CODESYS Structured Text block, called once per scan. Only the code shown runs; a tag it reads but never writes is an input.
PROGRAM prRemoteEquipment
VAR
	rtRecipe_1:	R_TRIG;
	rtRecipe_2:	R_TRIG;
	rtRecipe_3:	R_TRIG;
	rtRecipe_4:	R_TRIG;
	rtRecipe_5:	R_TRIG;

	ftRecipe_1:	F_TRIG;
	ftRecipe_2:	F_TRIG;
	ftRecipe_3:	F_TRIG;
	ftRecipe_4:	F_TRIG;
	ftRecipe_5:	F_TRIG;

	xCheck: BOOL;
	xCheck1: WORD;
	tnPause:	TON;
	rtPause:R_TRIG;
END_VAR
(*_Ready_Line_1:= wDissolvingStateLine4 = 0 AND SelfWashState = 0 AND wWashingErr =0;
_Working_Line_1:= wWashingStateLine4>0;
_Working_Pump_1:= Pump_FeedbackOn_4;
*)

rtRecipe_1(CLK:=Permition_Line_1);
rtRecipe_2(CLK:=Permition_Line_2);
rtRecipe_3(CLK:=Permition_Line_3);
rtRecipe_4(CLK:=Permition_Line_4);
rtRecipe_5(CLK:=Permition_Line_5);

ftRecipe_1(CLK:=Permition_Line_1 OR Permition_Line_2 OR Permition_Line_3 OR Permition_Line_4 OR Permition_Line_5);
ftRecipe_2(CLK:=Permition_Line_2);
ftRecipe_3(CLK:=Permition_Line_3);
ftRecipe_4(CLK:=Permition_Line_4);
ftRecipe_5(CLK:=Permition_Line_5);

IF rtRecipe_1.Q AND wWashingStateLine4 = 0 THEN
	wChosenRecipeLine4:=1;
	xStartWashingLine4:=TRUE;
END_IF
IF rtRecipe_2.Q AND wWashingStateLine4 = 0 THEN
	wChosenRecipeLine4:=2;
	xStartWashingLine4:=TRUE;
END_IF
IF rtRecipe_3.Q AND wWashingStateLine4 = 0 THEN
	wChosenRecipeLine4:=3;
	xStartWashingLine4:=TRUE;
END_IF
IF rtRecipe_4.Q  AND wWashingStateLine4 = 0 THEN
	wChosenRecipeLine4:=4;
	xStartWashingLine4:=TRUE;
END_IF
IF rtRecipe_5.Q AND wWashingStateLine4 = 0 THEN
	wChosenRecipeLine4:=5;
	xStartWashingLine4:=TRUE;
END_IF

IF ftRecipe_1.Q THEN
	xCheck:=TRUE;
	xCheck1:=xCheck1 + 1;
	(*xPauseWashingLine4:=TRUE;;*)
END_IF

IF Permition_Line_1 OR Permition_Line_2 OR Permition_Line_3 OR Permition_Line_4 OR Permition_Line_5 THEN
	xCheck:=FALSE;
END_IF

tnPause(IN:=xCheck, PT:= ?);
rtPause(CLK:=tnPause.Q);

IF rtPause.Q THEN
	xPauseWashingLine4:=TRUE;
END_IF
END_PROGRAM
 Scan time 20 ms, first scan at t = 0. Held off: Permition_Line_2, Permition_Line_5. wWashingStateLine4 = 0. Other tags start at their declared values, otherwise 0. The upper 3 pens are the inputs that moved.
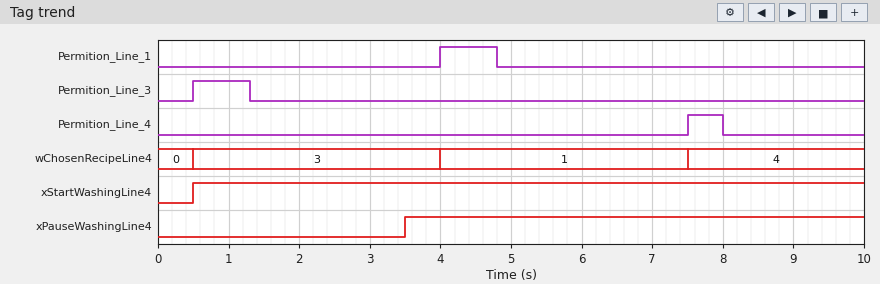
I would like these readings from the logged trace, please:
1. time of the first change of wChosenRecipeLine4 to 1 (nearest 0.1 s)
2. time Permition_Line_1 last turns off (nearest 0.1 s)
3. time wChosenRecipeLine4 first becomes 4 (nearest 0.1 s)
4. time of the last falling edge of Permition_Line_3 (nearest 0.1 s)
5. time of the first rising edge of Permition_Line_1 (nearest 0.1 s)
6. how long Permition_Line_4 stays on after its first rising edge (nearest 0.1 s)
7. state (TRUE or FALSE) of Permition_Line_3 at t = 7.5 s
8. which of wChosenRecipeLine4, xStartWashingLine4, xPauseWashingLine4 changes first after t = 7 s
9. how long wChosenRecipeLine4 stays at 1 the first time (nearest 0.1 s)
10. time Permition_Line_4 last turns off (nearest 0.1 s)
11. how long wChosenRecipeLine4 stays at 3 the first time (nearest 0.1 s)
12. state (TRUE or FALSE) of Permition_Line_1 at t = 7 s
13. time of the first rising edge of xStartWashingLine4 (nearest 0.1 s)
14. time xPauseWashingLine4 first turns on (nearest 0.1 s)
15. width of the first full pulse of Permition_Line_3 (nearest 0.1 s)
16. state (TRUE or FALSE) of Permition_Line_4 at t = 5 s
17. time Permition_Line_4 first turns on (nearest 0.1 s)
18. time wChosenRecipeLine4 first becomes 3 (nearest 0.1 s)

4.0 s
4.8 s
7.5 s
1.3 s
4.0 s
0.5 s
FALSE
wChosenRecipeLine4
3.5 s
8.0 s
3.5 s
FALSE
0.5 s
3.5 s
0.8 s
FALSE
7.5 s
0.5 s
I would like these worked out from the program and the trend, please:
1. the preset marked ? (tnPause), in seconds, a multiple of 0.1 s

2.2 s
